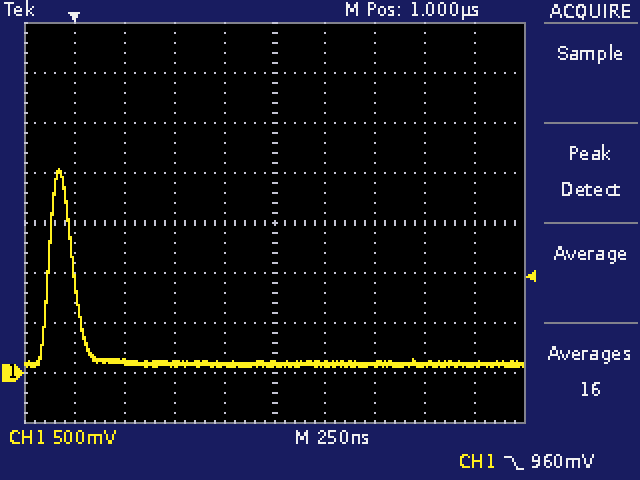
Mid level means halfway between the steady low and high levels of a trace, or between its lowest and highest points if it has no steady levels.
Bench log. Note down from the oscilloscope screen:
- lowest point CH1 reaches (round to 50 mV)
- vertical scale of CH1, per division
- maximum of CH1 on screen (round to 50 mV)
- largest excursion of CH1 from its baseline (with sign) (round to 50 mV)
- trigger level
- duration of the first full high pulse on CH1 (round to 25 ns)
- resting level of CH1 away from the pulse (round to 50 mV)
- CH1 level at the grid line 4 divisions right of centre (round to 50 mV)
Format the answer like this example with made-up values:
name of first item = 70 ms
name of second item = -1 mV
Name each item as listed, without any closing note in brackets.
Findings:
lowest point CH1 reaches = 50 mV
vertical scale of CH1, per division = 500 mV
maximum of CH1 on screen = 2.05 V
largest excursion of CH1 from its baseline (with sign) = +1.95 V
trigger level = 960 mV
duration of the first full high pulse on CH1 = 125 ns
resting level of CH1 away from the pulse = 100 mV
CH1 level at the grid line 4 divisions right of centre = 100 mV
